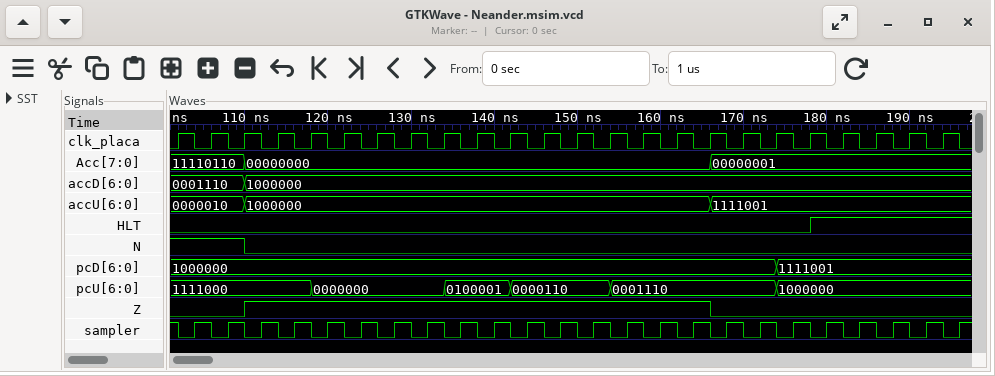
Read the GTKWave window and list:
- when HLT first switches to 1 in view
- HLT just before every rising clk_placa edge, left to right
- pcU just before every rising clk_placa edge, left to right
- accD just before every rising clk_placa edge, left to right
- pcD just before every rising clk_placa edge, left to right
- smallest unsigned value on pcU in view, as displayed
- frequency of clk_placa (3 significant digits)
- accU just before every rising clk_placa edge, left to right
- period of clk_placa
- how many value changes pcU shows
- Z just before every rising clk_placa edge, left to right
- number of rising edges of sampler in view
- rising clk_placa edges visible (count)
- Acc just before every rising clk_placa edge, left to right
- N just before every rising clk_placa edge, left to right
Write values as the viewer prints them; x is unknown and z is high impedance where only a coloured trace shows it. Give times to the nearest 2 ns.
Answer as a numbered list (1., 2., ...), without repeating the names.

1. 178 ns
2. 0 0 0 0 0 0 0 0 0 0 0 0 0 0 0 0 0 0 0 0 1 1 1 1
3. 1111000, 1111000, 1111000, 1111000, 1111000, 0000000, 0000000, 0000000, 0000000, 0100001, 0100001, 0000110, 0000110, 0000110, 0001110, 0001110, 0001110, 0001110, 0001110, 1000000, 1000000, 1000000, 1000000, 1000000
4. 0001110, 0001110, 0001110, 1000000, 1000000, 1000000, 1000000, 1000000, 1000000, 1000000, 1000000, 1000000, 1000000, 1000000, 1000000, 1000000, 1000000, 1000000, 1000000, 1000000, 1000000, 1000000, 1000000, 1000000
5. 1000000, 1000000, 1000000, 1000000, 1000000, 1000000, 1000000, 1000000, 1000000, 1000000, 1000000, 1000000, 1000000, 1000000, 1000000, 1000000, 1000000, 1000000, 1000000, 1111001, 1111001, 1111001, 1111001, 1111001
6. 0000000
7. 250 MHz
8. 0000010, 0000010, 0000010, 1000000, 1000000, 1000000, 1000000, 1000000, 1000000, 1000000, 1000000, 1000000, 1000000, 1000000, 1000000, 1000000, 1000000, 1111001, 1111001, 1111001, 1111001, 1111001, 1111001, 1111001
9. 4 ns
10. 5
11. 0 0 0 1 1 1 1 1 1 1 1 1 1 1 1 1 1 0 0 0 0 0 0 0
12. 24
13. 24
14. 11110110, 11110110, 11110110, 00000000, 00000000, 00000000, 00000000, 00000000, 00000000, 00000000, 00000000, 00000000, 00000000, 00000000, 00000000, 00000000, 00000000, 00000001, 00000001, 00000001, 00000001, 00000001, 00000001, 00000001
15. 1 1 1 0 0 0 0 0 0 0 0 0 0 0 0 0 0 0 0 0 0 0 0 0
